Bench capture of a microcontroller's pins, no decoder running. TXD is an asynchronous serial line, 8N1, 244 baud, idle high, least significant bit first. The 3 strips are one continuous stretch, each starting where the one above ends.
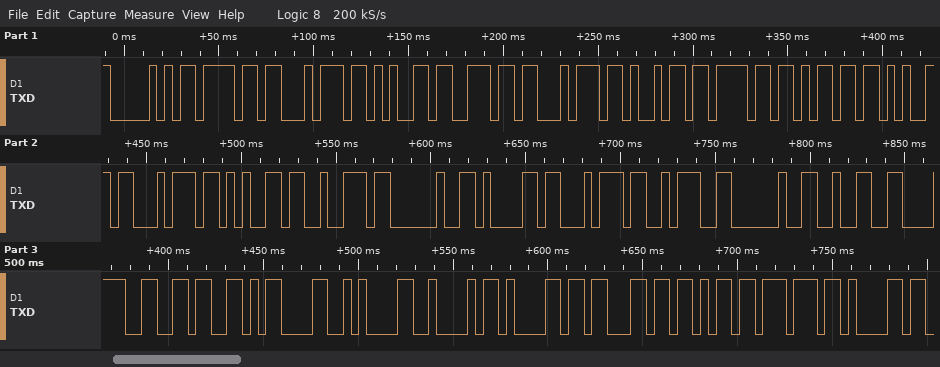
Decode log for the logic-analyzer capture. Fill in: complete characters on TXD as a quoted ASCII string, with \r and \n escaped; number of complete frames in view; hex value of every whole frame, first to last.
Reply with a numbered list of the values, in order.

1. "Potentiometer at: 286\r\nBackwa"
2. 29
3. 50 6F 74 65 6E 74 69 6F 6D 65 74 65 72 20 61 74 3A 20 32 38 36 0D 0A 42 61 63 6B 77 61
